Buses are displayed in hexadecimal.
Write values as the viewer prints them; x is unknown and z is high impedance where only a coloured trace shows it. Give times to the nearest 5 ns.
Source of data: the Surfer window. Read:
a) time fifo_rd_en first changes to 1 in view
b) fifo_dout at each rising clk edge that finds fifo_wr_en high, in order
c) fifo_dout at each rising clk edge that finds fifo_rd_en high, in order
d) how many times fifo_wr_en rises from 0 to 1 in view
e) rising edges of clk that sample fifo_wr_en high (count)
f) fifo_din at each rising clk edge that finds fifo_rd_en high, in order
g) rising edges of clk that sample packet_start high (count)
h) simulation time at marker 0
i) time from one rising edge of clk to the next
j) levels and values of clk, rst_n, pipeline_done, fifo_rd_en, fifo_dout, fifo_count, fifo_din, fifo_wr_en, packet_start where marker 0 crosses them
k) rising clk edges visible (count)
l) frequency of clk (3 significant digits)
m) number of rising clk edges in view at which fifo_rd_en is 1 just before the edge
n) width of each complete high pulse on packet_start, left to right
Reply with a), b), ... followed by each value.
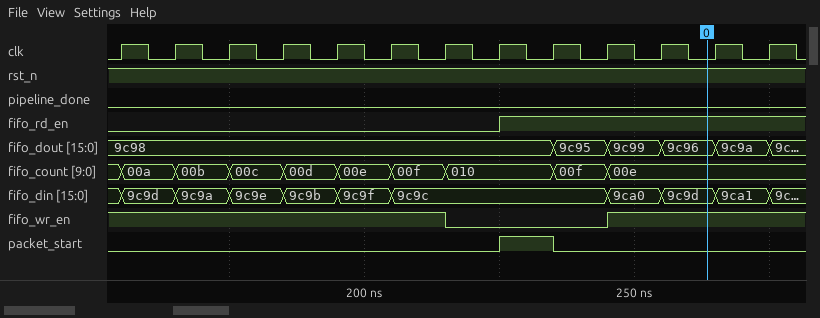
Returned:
a) 225 ns
b) 9c98, 9c98, 9c98, 9c98, 9c98, 9c98, 9c98, 9c99, 9c96, 9c9a
c) 9c98, 9c95, 9c99, 9c96, 9c9a
d) 1
e) 10
f) 9c9c, 9c9c, 9ca0, 9c9d, 9ca1
g) 1
h) 265 ns
i) 10 ns
j) clk=0, rst_n=1, pipeline_done=0, fifo_rd_en=1, fifo_dout=9c96, fifo_count=00e, fifo_din=9c9d, fifo_wr_en=1, packet_start=0
k) 13
l) 100 MHz
m) 5
n) 10 ns
